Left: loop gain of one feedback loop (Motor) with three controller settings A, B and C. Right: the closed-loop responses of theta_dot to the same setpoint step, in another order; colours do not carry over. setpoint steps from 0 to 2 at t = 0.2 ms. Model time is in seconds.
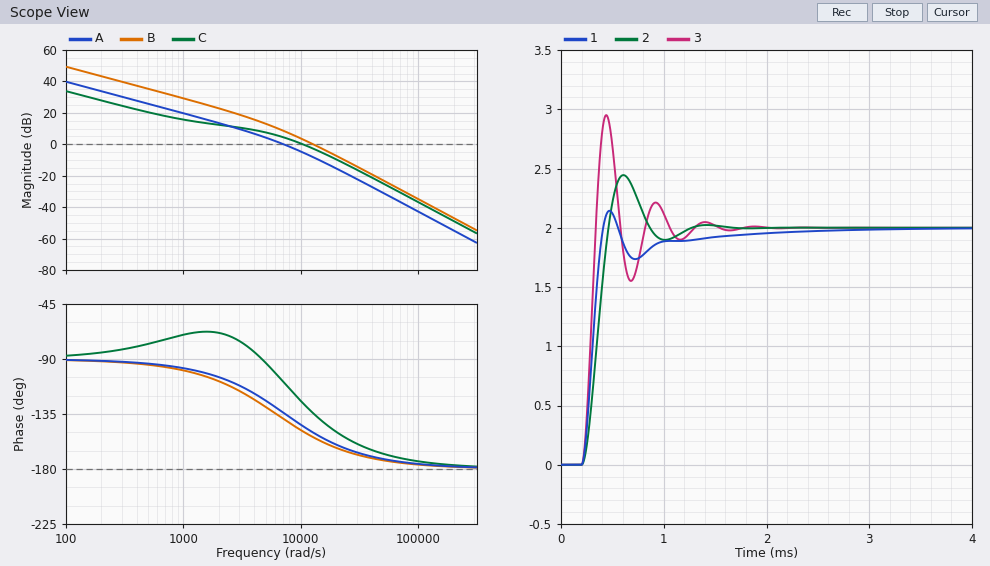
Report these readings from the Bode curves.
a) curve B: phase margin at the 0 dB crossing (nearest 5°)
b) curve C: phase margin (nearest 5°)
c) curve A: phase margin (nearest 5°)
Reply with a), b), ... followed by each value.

a) 25°
b) 55°
c) 45°
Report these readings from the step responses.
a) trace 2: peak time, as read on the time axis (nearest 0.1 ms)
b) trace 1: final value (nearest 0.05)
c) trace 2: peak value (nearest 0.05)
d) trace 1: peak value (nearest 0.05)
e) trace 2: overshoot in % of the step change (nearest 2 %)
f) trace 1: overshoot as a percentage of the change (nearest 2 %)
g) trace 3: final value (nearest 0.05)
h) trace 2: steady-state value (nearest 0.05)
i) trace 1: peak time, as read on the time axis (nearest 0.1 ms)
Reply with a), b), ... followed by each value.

a) 0.6 ms
b) 2.00
c) 2.45
d) 2.15
e) 22 %
f) 8 %
g) 2.00
h) 2.00
i) 0.5 ms
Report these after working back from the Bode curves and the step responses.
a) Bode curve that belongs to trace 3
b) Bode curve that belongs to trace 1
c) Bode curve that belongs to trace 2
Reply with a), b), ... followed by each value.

a) B
b) C
c) A
